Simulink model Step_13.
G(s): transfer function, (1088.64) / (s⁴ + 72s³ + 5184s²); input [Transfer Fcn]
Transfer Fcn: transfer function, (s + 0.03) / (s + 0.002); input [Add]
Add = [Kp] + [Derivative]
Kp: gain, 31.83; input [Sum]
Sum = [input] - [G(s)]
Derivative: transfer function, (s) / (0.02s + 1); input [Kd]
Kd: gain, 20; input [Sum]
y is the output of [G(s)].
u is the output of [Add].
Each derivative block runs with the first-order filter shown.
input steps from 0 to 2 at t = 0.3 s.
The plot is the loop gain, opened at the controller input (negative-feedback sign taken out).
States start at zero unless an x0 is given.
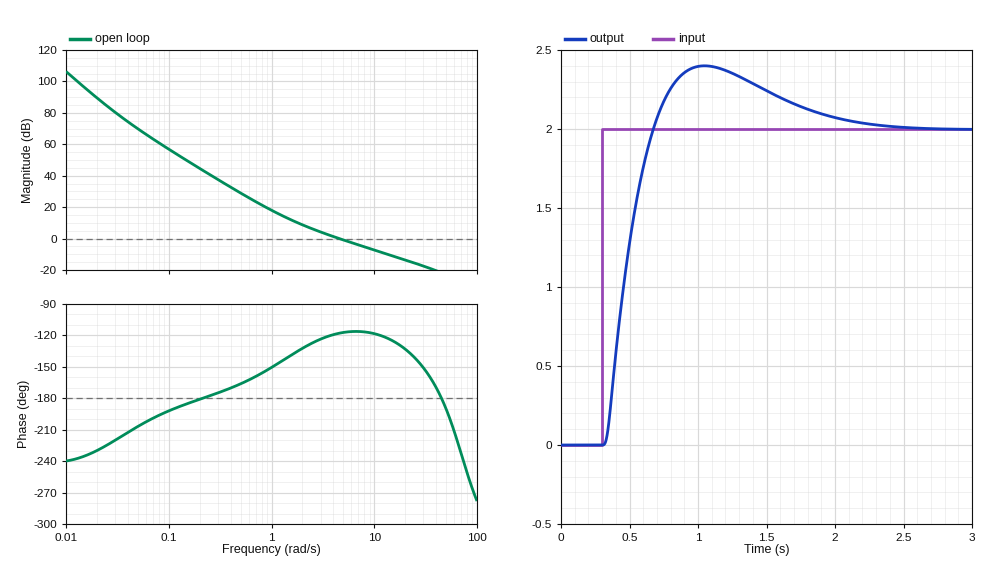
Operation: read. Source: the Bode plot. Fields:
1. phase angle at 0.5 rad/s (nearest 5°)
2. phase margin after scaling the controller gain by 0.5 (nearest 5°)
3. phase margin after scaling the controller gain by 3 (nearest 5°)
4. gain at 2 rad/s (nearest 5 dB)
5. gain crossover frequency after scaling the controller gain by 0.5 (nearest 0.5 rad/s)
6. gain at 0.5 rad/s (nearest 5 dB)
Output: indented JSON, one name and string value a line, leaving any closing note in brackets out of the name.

{
  "phase angle at 0.5 rad/s": "-165°",
  "phase margin after scaling the controller gain by 0.5": "55°",
  "phase margin after scaling the controller gain by 3": "60°",
  "gain at 2 rad/s": "10 dB",
  "gain crossover frequency after scaling the controller gain by 0.5": "2.5 rad/s",
  "gain at 0.5 rad/s": "30 dB"
}
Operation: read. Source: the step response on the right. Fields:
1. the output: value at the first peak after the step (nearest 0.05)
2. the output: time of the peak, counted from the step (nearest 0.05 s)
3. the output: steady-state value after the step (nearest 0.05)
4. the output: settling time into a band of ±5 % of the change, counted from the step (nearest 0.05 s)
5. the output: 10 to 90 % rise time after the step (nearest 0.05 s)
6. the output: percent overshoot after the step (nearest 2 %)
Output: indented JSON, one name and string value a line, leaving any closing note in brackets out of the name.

{
  "the output: value at the first peak after the step": "2.40",
  "the output: time of the peak, counted from the step": "0.75 s",
  "the output: steady-state value after the step": "2.00",
  "the output: settling time into a band of ±5 % of the change, counted from the step": "1.60 s",
  "the output: 10 to 90 % rise time after the step": "0.25 s",
  "the output: percent overshoot after the step": "20 %"
}
